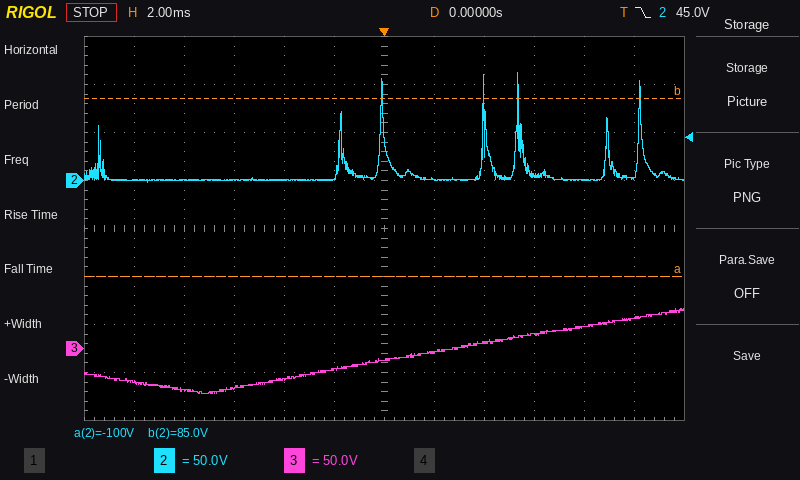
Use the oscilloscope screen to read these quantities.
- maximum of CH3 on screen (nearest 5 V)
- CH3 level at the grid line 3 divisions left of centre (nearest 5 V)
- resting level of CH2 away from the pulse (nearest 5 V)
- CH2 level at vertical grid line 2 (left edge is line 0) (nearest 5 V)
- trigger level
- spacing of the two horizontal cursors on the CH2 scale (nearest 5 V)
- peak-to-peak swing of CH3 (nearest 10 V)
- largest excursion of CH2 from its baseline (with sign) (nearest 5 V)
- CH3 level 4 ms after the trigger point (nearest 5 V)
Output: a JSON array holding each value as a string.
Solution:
["40 V", "-40 V", "0 V", "0 V", "45.0 V", "185 V", "90 V", "+110 V", "5 V"]
